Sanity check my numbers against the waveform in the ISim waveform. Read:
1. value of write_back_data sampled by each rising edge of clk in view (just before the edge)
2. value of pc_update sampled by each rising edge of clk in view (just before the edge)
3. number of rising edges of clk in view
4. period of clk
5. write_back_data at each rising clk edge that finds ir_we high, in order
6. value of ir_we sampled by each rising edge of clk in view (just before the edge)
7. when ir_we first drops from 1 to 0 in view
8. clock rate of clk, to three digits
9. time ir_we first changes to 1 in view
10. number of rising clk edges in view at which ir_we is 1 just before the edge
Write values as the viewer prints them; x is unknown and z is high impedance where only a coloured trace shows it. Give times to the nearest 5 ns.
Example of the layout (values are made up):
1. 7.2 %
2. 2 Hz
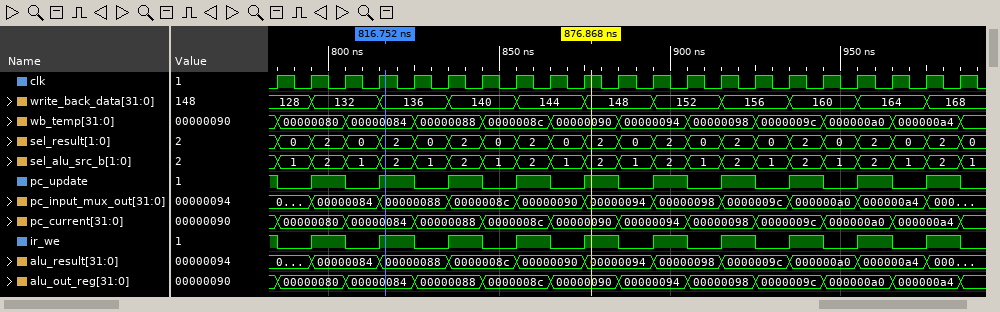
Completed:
1. 128, 128, 132, 132, 136, 136, 140, 140, 144, 144, 148, 148, 152, 152, 156, 156, 160, 160, 164, 164, 168
2. 1 0 1 0 1 0 1 0 1 0 1 0 1 0 1 0 1 0 1 0 1
3. 21
4. 10 ns
5. 128, 132, 136, 140, 144, 148, 152, 156, 160, 164, 168
6. 1 0 1 0 1 0 1 0 1 0 1 0 1 0 1 0 1 0 1 0 1
7. 785 ns
8. 100 MHz
9. 795 ns
10. 11
